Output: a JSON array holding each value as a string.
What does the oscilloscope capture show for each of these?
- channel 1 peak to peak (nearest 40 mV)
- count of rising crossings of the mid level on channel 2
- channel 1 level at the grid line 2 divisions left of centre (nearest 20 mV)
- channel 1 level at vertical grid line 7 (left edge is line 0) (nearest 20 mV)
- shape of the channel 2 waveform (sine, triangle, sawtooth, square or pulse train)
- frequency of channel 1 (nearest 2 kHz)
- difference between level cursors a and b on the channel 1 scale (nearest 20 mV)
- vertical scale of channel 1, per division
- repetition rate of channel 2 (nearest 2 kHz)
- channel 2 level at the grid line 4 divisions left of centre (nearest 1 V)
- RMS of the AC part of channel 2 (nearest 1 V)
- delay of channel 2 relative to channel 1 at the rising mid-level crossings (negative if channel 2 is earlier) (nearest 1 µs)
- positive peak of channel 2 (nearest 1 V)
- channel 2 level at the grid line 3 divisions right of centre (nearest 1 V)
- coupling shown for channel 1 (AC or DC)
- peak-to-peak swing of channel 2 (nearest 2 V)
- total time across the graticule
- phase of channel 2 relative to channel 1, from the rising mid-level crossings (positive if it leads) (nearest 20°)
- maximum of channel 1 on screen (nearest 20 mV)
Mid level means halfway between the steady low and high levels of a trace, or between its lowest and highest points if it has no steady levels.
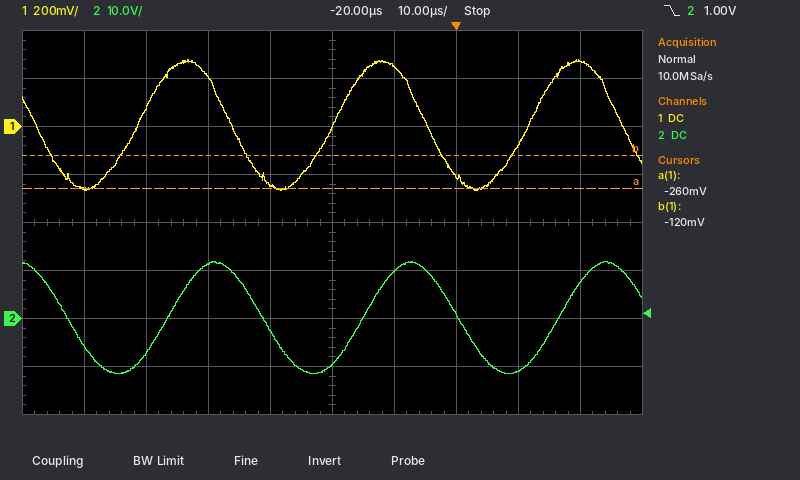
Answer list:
["560 mV", "3", "200 mV", "-200 mV", "sine", "32 kHz", "140 mV", "200 mV", "32 kHz", "-6 V", "8 V", "+5 µs", "12 V", "-11 V", "DC", "24 V", "100 µs", "-60°", "280 mV"]
